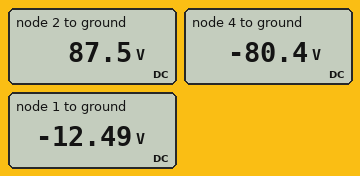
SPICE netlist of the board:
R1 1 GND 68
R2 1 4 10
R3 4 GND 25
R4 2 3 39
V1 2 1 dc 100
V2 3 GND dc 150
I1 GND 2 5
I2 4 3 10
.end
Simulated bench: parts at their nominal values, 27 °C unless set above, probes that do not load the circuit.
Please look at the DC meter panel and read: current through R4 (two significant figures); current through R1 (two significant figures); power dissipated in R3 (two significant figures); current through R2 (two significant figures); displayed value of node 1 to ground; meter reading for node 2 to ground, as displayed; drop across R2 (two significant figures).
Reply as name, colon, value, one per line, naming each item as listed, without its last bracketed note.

current through R4: 1.6 A
current through R1: 180 mA
power dissipated in R3: 260 W
current through R2: 6.8 A
displayed value of node 1 to ground: -12.49 V
meter reading for node 2 to ground, as displayed: 87.5 V
drop across R2: 68 V
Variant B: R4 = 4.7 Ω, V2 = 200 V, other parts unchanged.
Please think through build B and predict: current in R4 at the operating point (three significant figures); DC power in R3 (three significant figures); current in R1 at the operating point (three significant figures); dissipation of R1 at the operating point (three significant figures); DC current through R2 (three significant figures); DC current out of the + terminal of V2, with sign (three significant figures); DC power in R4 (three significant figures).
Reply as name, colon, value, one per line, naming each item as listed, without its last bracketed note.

current in R4 at the operating point: 5.38 A
DC power in R3: 13.0 W
current in R1 at the operating point: 1.10 A
dissipation of R1 at the operating point: 82.1 W
DC current through R2: 9.28 A
DC current out of the + terminal of V2, with sign: -4.62 A
DC power in R4: 136 W
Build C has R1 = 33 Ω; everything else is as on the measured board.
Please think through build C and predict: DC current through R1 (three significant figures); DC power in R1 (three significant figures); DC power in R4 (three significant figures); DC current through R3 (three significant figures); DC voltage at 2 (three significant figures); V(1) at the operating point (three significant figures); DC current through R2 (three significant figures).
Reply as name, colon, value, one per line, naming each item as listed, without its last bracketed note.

DC current through R1: 309 mA
DC power in R1: 3.14 W
DC power in R4: 92.9 W
DC current through R3: 3.15 A
DC voltage at 2: 89.8 V
V(1) at the operating point: -10.2 V
DC current through R2: 6.85 A
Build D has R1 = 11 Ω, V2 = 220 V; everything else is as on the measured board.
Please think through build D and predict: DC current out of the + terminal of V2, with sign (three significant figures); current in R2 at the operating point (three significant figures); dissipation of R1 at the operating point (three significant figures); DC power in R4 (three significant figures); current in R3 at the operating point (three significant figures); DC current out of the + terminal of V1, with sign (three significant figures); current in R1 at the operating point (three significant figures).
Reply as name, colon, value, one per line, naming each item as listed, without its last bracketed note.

DC current out of the + terminal of V2, with sign: -7.09 A
current in R2 at the operating point: 7.33 A
dissipation of R1 at the operating point: 3.77 W
DC power in R4: 331 W
current in R3 at the operating point: 2.67 A
DC current out of the + terminal of V1, with sign: -7.91 A
current in R1 at the operating point: 585 mA
